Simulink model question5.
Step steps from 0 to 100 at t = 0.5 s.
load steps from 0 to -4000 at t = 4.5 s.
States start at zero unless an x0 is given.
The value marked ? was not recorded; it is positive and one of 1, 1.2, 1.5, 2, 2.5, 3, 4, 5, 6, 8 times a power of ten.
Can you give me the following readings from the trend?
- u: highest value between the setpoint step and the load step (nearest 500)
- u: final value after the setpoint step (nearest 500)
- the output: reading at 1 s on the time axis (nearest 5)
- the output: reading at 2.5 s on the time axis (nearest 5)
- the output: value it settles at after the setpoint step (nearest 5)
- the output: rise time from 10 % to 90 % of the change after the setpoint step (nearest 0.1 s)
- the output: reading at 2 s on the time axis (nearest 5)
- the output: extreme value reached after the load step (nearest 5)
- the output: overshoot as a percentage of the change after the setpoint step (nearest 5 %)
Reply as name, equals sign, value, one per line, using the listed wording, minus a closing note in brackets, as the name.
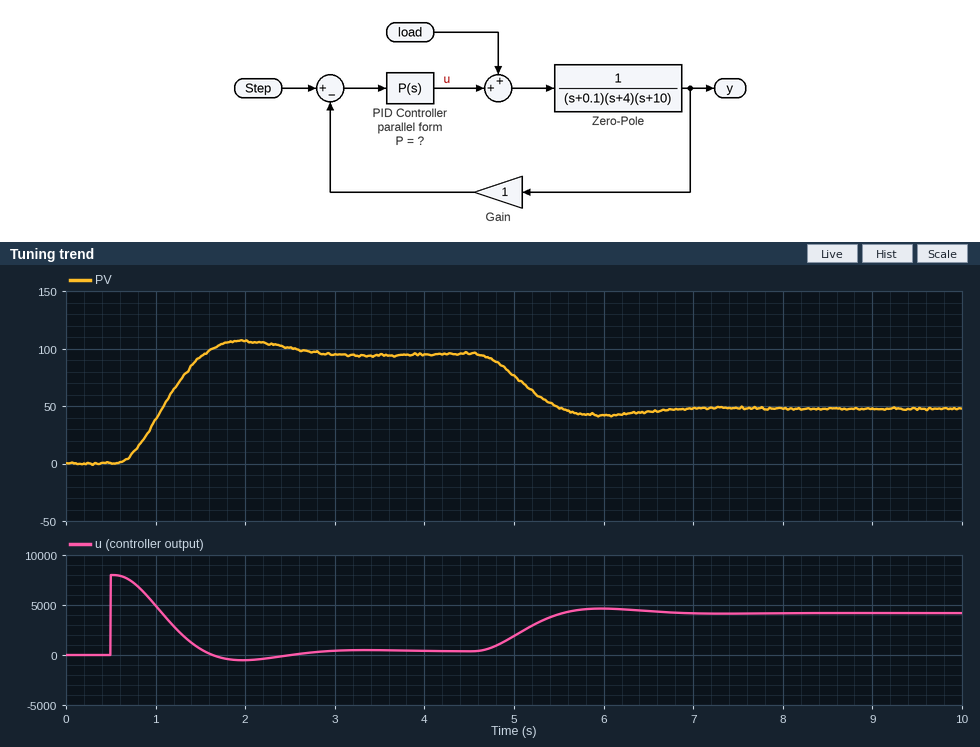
u: highest value between the setpoint step and the load step = 8000
u: final value after the setpoint step = 500
the output: reading at 1 s on the time axis = 40
the output: reading at 2.5 s on the time axis = 100
the output: value it settles at after the setpoint step = 95
the output: rise time from 10 % to 90 % of the change after the setpoint step = 0.7 s
the output: reading at 2 s on the time axis = 105
the output: extreme value reached after the load step = 40
the output: overshoot as a percentage of the change after the setpoint step = 10 %
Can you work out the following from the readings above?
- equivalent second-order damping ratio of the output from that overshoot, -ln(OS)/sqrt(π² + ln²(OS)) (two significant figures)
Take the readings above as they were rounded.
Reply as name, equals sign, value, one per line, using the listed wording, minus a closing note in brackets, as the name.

equivalent second-order damping ratio of the output from that overshoot, -ln(OS)/sqrt(π² + ln²(OS)) = 0.59
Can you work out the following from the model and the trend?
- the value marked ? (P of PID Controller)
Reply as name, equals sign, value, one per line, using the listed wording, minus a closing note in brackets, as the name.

the value marked ? = 80
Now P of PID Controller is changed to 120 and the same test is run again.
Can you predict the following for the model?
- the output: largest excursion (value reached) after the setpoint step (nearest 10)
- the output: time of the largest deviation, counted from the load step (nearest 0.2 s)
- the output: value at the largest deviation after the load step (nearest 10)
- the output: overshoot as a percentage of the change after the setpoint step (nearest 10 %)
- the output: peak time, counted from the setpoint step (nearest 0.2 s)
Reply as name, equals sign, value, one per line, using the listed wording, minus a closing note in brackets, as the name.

the output: largest excursion (value reached) after the setpoint step = 120
the output: time of the largest deviation, counted from the load step = 1.2 s
the output: value at the largest deviation after the load step = 60
the output: overshoot as a percentage of the change after the setpoint step = 20 %
the output: peak time, counted from the setpoint step = 1.2 s
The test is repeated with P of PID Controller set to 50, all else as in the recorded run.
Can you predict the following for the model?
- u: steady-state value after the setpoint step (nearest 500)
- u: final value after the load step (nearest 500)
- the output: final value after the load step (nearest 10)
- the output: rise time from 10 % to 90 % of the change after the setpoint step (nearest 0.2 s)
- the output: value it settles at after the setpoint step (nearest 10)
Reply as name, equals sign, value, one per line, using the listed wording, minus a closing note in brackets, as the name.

u: steady-state value after the setpoint step = 500
u: final value after the load step = 4000
the output: final value after the load step = 20
the output: rise time from 10 % to 90 % of the change after the setpoint step = 1.0 s
the output: value it settles at after the setpoint step = 90
